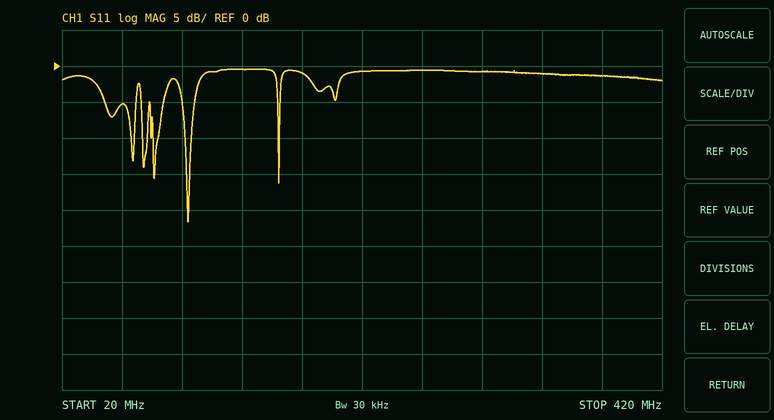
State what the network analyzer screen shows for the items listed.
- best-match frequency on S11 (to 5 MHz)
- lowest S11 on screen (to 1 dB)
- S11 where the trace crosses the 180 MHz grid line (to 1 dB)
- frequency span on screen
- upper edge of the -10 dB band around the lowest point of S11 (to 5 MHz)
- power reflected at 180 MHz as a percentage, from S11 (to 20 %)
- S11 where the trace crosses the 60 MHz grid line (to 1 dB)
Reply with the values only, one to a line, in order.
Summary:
105 MHz
-22 dB
-1 dB
400 MHz
105 MHz
80 %
-5 dB
